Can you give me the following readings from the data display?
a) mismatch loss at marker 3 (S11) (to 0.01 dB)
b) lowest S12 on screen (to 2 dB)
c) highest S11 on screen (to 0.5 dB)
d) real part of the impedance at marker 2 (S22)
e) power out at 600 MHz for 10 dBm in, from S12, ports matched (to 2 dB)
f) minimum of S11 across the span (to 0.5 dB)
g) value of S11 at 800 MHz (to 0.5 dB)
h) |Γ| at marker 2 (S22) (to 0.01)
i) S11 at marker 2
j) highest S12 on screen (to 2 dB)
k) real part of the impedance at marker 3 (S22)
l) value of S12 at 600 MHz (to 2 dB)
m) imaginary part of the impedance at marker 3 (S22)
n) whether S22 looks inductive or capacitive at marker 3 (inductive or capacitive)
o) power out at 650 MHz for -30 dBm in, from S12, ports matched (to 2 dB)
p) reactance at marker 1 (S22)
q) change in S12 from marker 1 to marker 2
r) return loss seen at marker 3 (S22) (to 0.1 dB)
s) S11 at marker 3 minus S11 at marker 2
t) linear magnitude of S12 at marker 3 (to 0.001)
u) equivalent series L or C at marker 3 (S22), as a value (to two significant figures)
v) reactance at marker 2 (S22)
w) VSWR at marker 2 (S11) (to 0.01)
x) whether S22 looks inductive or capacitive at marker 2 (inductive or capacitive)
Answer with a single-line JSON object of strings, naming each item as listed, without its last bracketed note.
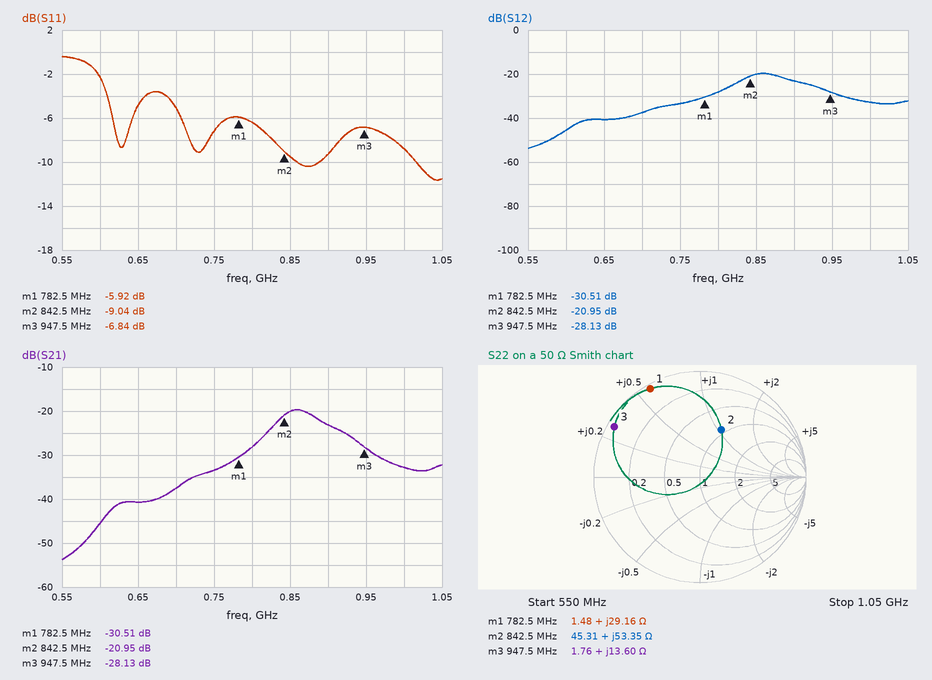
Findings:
{"mismatch loss at marker 3 (S11)": "1.01 dB", "lowest S12 on screen": "-54 dB", "highest S11 on screen": "-0.5 dB", "real part of the impedance at marker 2": "45.31 Ω", "power out at 600 MHz for 10 dBm in, from S12, ports matched": "-36 dBm", "minimum of S11 across the span": "-11.5 dB", "value of S11 at 800 MHz": "-6.5 dB", "|Γ| at marker 2 (S22)": "0.49", "S11 at marker 2": "-9.04 dB", "highest S12 on screen": "-20 dB", "real part of the impedance at marker 3": "1.76 Ω", "value of S12 at 600 MHz": "-46 dB", "imaginary part of the impedance at marker 3": "+13.60 Ω", "whether S22 looks inductive or capacitive at marker 3": "inductive", "power out at 650 MHz for -30 dBm in, from S12, ports matched": "-70 dBm", "reactance at marker 1": "+29.16 Ω", "change in S12 from marker 1 to marker 2": "9.56 dB", "return loss seen at marker 3 (S22)": "0.6 dB", "S11 at marker 3 minus S11 at marker 2": "2.20 dB", "linear magnitude of S12 at marker 3": "0.039", "equivalent series L or C at marker 3 (S22), as a value": "2.3 nH", "reactance at marker 2": "+53.35 Ω", "VSWR at marker 2 (S11)": "2.09", "whether S22 looks inductive or capacitive at marker 2": "inductive"}
